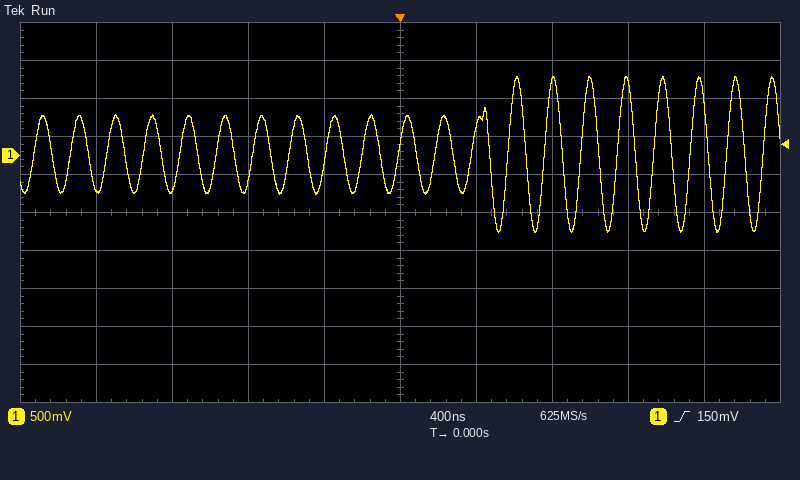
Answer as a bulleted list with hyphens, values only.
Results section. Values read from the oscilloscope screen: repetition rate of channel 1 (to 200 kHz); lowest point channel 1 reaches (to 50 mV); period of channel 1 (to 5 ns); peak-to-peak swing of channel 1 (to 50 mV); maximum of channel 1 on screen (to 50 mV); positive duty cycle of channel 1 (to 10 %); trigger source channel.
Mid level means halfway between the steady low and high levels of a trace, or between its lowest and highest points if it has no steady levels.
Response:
- 5.2 MHz
- -1.00 V
- 190 ns
- 2.05 V
- 1.05 V
- 50 %
- channel 1
